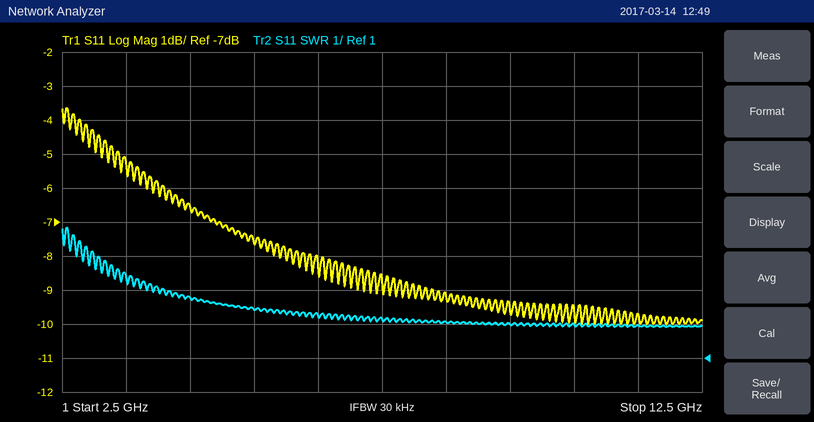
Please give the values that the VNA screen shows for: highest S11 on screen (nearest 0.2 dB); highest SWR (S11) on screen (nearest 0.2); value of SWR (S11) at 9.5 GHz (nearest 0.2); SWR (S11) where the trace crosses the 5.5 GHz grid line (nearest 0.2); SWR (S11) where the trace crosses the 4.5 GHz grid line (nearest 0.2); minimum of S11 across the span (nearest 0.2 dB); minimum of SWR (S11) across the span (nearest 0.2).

-3.6 dB
4.8
2.0
2.4
2.8
-10.0 dB
2.0
